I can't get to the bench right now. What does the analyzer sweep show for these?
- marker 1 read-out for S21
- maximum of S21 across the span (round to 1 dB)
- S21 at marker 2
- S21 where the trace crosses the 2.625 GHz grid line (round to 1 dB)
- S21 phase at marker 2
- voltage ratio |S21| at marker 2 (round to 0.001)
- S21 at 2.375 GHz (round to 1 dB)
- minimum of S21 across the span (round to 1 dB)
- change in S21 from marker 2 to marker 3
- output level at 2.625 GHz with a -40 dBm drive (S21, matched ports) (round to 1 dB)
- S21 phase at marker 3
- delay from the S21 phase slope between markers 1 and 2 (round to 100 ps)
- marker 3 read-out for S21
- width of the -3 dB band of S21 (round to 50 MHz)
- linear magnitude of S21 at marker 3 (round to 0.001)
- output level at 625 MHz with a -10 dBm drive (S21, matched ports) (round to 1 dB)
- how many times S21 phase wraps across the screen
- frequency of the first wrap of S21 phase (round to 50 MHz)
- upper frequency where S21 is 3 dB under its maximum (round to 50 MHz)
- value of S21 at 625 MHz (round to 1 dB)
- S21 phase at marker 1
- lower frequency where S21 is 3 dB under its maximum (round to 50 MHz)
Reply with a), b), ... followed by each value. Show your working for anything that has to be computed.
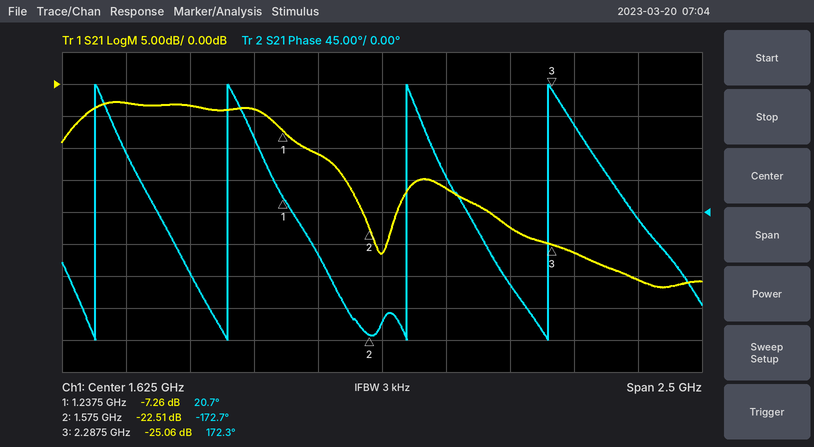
a) -7.26 dB
b) -3 dB
c) -22.51 dB
d) -31 dB
e) -172.7°
f) 10^(-22.51/20) ≈ 0.075
g) -26 dB
h) -32 dB
i) -25.06 − (-22.51) = -2.55 dB
j) -40 dBm + (-31 dB) = -71 dBm
k) 172.3°
l) −(-172.7° − (20.7°))/(360° × 337.5 MHz) ≈ 1.6 ns
m) -25.06 dB
n) 1.20 GHz − 450 MHz = 750 MHz
o) 10^(-25.06/20) ≈ 0.056
p) -10 dBm + (-3 dB) = -13 dBm
q) 4
r) 500 MHz
s) 1.20 GHz
t) -3 dB
u) 20.7°
v) 450 MHz
